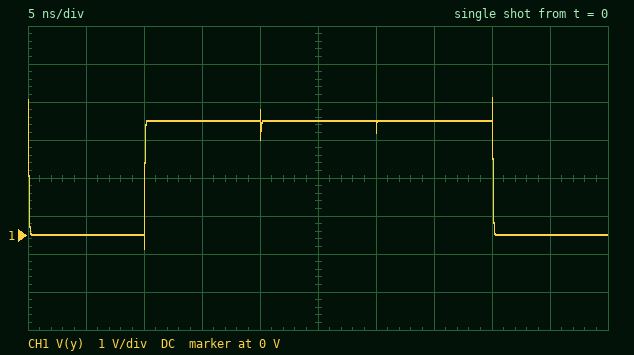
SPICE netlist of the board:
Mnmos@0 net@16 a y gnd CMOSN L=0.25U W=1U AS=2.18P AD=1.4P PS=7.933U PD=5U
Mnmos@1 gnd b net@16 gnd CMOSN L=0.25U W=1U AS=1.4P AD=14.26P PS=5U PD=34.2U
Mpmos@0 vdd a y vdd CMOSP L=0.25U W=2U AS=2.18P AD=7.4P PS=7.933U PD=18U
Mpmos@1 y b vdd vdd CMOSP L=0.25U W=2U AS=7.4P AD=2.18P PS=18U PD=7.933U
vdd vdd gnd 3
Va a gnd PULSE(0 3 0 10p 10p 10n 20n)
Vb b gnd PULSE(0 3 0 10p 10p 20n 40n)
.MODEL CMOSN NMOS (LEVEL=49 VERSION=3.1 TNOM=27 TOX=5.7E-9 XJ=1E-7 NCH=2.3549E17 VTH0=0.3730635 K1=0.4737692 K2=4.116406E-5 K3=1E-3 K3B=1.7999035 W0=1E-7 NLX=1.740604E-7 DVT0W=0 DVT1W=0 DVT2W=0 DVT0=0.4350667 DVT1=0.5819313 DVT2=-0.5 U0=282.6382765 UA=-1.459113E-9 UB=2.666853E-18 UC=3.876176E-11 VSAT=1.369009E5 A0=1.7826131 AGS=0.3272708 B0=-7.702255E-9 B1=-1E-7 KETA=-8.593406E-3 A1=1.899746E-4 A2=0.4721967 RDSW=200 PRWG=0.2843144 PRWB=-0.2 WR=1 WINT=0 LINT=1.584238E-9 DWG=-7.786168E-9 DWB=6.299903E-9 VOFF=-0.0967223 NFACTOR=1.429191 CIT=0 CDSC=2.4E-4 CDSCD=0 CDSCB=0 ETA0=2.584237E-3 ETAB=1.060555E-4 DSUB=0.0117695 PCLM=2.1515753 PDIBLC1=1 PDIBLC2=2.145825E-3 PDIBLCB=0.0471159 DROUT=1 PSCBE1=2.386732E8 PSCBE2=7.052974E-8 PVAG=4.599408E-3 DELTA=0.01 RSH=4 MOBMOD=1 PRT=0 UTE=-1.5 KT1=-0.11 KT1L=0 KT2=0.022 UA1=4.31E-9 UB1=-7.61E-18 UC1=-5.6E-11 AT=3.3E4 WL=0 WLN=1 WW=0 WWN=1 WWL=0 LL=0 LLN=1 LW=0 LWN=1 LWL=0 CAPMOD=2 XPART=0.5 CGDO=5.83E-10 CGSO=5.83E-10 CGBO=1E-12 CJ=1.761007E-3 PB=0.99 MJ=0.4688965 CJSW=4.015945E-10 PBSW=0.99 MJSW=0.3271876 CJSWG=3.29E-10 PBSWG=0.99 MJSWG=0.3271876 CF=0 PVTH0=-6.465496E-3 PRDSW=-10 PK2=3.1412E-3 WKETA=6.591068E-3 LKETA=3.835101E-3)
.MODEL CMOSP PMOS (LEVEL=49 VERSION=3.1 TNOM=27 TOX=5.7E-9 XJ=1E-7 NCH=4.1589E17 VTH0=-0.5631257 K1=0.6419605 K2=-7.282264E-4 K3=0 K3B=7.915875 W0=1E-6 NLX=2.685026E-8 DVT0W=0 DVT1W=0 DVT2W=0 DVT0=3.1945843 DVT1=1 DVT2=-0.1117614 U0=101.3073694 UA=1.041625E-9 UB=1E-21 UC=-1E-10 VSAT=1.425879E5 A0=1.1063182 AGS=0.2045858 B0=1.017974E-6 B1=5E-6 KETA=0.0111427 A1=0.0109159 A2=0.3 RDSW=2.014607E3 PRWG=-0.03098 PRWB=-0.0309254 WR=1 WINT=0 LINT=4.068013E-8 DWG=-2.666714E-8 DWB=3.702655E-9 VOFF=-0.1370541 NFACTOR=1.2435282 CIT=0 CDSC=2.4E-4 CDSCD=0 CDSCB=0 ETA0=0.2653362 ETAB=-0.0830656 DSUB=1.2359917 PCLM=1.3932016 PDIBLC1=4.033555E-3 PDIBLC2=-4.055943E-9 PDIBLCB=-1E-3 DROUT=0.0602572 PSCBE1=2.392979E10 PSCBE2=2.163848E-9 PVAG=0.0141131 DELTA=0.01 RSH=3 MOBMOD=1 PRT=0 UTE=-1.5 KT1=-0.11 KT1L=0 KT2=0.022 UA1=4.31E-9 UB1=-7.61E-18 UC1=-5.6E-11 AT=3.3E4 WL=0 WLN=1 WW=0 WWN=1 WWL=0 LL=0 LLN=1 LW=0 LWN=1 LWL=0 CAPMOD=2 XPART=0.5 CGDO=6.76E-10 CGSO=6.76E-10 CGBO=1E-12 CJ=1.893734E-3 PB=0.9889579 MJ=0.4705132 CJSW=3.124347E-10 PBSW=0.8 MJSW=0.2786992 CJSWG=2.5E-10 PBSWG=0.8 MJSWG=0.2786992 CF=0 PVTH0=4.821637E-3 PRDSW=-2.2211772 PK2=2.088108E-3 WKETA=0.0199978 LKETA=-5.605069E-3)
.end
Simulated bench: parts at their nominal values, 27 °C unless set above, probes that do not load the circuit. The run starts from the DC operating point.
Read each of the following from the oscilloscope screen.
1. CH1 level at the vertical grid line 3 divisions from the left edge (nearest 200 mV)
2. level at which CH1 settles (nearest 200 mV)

3.0 V
0 V
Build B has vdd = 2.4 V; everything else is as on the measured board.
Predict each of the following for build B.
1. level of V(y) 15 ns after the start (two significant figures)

2.4 V
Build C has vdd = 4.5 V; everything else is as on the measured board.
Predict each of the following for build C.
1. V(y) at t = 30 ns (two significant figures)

4.5 V
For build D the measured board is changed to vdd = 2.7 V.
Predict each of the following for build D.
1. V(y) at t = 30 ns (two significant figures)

2.7 V
